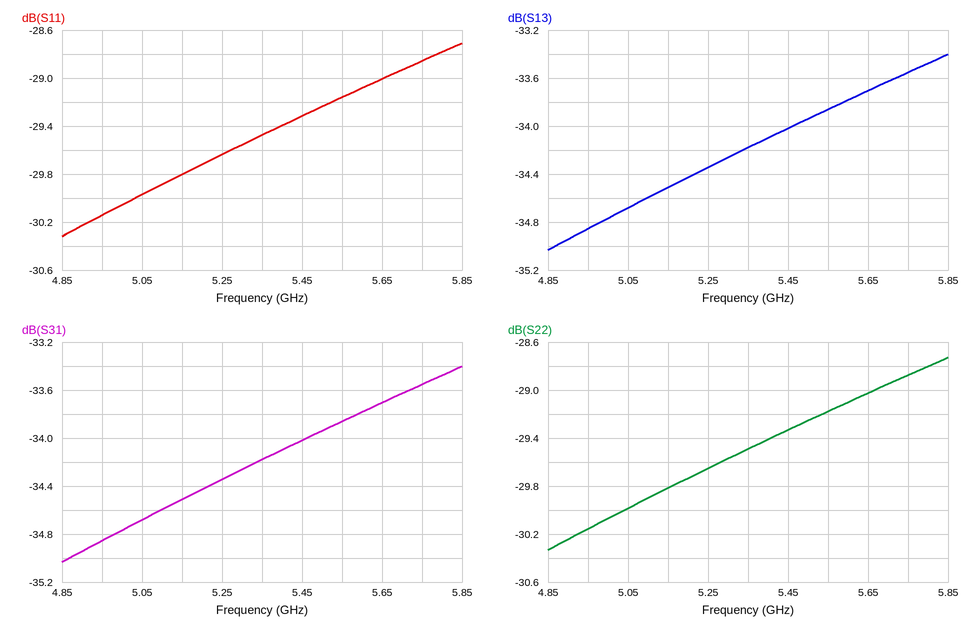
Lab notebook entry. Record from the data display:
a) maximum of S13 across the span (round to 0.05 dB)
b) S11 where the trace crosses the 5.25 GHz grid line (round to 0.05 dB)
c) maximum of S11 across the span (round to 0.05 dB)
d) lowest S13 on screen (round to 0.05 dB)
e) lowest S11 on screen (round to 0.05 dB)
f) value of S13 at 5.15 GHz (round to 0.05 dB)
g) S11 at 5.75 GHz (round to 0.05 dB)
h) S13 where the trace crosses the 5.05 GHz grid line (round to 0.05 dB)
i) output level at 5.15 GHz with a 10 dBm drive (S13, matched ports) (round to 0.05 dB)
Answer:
-33.40 dB
-29.65 dB
-28.70 dB
-35.05 dB
-30.30 dB
-34.50 dB
-28.85 dB
-34.70 dB
-24.50 dBm
